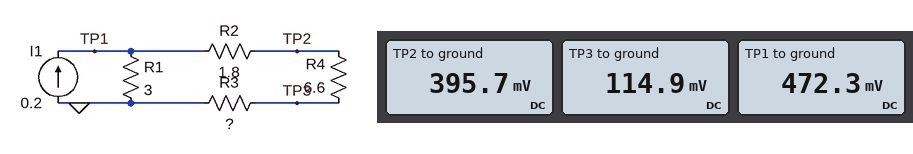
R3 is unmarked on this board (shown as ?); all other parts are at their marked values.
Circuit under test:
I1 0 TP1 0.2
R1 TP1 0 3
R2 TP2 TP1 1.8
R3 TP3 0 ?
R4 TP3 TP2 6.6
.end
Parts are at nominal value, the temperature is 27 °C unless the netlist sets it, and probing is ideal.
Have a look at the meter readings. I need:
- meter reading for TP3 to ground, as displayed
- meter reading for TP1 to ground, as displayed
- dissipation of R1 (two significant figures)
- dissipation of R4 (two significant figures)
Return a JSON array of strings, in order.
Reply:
["114.9 mV", "472.3 mV", "74 mW", "12 mW"]
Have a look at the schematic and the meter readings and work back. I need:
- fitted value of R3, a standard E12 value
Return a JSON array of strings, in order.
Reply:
["2.7 Ω"]
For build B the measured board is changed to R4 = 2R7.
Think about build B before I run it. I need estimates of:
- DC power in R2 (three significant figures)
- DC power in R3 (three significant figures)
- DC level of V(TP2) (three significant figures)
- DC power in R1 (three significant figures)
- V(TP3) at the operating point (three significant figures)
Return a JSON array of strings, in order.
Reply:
["6.23 mW", "9.34 mW", "318 mV", "59.8 mW", "159 mV"]
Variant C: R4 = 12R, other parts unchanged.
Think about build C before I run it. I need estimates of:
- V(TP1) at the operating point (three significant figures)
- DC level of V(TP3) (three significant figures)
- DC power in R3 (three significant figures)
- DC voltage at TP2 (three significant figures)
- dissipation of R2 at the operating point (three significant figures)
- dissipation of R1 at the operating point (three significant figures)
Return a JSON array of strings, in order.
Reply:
["508 mV", "83.1 mV", "2.56 mW", "452 mV", "1.70 mW", "85.9 mW"]
